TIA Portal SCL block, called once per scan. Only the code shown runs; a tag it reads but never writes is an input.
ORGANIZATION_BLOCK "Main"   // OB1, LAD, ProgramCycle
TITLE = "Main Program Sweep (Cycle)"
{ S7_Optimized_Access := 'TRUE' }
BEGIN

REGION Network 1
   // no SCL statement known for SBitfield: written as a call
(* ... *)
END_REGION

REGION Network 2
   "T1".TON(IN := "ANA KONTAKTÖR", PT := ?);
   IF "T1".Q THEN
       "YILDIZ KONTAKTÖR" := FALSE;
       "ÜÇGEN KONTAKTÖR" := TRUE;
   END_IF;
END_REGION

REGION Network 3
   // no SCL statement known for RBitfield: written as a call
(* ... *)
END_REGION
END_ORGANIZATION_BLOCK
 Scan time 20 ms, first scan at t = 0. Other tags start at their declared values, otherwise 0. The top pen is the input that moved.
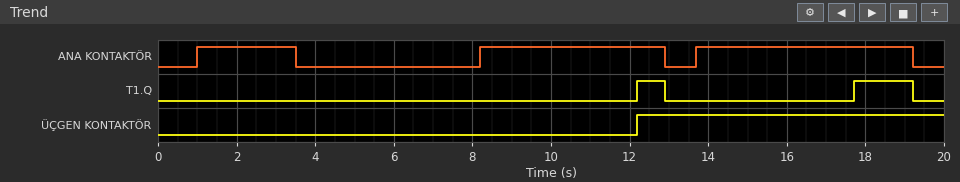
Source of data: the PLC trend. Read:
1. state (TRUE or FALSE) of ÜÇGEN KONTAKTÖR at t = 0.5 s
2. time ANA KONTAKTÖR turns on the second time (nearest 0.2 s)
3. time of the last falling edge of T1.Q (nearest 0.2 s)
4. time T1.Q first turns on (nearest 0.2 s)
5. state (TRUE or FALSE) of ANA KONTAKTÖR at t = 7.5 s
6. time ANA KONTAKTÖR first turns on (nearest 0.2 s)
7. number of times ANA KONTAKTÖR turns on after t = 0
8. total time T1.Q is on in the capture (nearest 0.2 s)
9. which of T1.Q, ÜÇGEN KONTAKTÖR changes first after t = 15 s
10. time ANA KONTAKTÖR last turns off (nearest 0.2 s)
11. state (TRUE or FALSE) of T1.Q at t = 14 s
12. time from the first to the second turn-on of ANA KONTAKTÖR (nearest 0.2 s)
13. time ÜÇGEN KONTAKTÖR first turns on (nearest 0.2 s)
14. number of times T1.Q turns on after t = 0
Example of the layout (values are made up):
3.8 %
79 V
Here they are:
FALSE
8.2 s
19.2 s
12.2 s
FALSE
1.0 s
3
2.2 s
T1.Q
19.2 s
FALSE
7.2 s
12.2 s
2
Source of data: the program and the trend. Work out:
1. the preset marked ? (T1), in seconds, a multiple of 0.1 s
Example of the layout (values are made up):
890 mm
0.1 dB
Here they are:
4.0 s
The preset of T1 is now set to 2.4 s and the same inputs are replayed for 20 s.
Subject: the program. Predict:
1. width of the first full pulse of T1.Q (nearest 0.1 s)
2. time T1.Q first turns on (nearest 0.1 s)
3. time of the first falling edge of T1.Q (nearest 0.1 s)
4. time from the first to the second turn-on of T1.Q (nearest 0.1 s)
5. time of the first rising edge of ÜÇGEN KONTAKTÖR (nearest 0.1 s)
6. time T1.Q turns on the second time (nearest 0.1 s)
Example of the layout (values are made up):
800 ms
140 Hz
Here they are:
0.1 s
3.4 s
3.5 s
7.2 s
3.4 s
10.6 s
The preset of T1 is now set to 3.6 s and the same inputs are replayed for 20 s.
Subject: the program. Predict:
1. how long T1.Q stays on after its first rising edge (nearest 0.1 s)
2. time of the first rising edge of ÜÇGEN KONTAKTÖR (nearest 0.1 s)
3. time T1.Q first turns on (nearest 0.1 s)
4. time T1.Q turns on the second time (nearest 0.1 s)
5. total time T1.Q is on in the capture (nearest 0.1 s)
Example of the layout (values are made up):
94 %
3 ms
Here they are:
1.1 s
11.8 s
11.8 s
17.3 s
3.0 s
